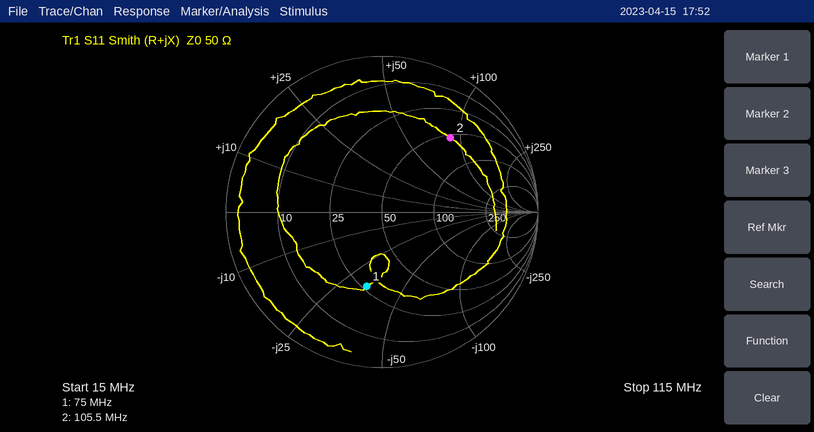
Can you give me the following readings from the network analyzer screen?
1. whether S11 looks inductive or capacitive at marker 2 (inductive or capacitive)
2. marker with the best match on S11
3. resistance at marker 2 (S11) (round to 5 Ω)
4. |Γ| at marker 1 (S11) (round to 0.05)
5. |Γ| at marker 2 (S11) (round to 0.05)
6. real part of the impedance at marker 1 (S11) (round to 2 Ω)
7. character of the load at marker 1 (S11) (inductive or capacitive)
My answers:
inductive
marker 1
55 Ω
0.50
0.65
26 Ω
capacitive
